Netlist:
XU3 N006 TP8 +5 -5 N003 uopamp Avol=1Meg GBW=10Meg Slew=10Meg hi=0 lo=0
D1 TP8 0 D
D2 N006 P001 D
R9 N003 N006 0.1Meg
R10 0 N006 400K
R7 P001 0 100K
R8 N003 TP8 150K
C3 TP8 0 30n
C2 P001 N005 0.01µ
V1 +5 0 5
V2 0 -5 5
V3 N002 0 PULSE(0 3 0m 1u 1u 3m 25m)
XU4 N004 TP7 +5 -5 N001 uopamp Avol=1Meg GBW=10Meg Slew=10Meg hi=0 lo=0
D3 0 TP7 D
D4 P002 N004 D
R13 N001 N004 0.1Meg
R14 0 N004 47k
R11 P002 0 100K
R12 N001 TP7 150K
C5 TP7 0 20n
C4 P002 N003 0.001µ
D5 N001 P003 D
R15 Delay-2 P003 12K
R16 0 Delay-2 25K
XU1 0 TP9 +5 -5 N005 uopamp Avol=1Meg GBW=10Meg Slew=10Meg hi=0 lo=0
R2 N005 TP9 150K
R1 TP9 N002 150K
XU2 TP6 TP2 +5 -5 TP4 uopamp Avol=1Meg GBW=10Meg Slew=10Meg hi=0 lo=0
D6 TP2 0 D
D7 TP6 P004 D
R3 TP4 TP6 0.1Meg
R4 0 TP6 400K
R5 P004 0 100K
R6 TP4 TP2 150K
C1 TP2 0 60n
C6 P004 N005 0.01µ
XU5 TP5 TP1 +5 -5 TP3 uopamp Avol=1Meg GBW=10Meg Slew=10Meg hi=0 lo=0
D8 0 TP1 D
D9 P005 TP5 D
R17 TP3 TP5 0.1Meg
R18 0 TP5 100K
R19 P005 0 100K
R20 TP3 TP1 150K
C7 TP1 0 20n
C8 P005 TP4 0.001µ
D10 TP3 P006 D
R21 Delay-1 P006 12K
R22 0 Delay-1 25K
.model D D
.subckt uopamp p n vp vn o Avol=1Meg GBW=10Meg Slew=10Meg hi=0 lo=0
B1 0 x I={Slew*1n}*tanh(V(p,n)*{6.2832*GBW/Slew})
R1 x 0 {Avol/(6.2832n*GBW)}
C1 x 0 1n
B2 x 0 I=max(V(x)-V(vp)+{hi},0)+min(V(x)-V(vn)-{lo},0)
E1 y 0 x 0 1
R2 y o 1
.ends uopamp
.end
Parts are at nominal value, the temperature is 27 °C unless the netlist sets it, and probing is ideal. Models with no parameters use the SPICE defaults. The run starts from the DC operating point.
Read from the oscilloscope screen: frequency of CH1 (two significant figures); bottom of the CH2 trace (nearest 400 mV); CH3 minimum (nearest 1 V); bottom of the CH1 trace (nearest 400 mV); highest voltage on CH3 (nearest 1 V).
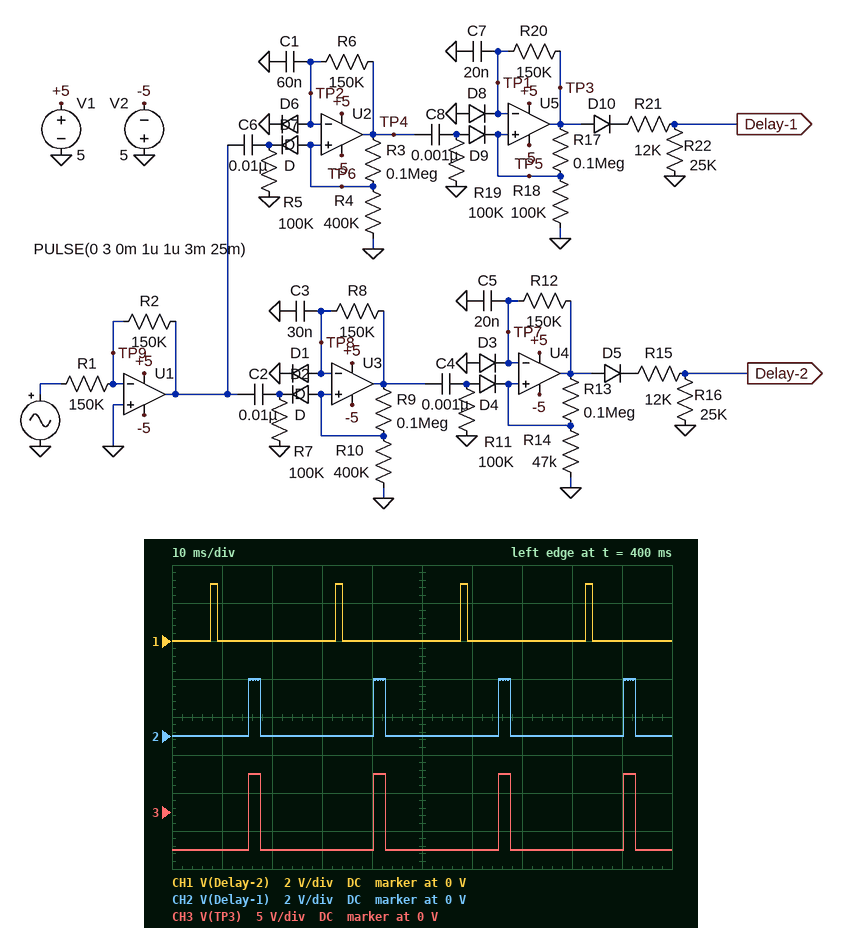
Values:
40 Hz
0 V
-5 V
0 V
5 V
